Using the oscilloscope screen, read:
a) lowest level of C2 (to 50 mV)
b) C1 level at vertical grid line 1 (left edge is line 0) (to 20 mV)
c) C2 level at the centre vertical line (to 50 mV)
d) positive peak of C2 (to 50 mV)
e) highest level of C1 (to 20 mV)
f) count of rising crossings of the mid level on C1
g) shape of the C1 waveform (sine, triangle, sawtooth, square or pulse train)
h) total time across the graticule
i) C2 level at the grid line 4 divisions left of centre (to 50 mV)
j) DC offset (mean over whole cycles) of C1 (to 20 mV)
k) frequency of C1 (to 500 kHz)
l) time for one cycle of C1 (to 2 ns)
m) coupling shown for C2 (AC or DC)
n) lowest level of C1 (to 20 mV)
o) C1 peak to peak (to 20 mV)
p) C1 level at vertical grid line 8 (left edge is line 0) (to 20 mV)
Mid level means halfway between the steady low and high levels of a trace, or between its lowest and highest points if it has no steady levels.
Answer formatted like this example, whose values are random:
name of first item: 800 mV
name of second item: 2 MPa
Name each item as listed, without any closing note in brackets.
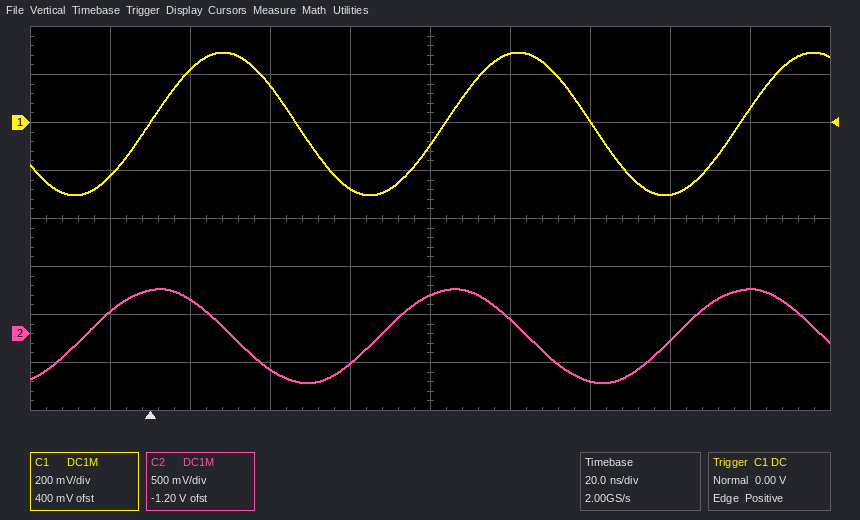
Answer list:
lowest level of C2: -500 mV
C1 level at vertical grid line 1 (left edge is line 0): -220 mV
C2 level at the centre vertical line: 400 mV
positive peak of C2: 450 mV
highest level of C1: 300 mV
count of rising crossings of the mid level on C1: 3
shape of the C1 waveform: sine
total time across the graticule: 200 ns
C2 level at the grid line 4 divisions left of centre: 250 mV
DC offset (mean over whole cycles) of C1: 0 mV
frequency of C1: 13.5 MHz
time for one cycle of C1: 74 ns
coupling shown for C2: DC
lowest level of C1: -300 mV
C1 peak to peak: 600 mV
C1 level at vertical grid line 8 (left edge is line 0): -300 mV
